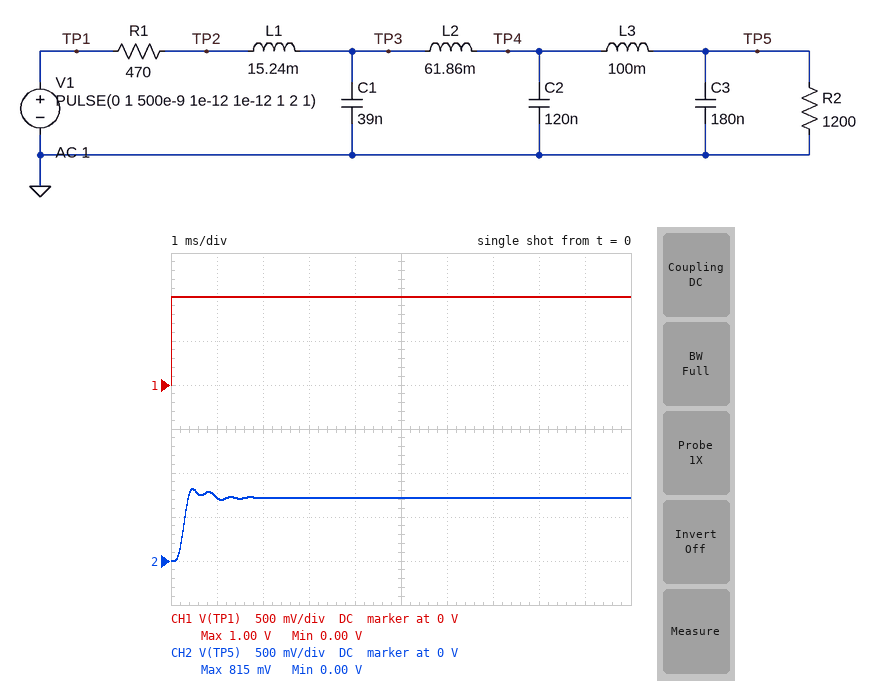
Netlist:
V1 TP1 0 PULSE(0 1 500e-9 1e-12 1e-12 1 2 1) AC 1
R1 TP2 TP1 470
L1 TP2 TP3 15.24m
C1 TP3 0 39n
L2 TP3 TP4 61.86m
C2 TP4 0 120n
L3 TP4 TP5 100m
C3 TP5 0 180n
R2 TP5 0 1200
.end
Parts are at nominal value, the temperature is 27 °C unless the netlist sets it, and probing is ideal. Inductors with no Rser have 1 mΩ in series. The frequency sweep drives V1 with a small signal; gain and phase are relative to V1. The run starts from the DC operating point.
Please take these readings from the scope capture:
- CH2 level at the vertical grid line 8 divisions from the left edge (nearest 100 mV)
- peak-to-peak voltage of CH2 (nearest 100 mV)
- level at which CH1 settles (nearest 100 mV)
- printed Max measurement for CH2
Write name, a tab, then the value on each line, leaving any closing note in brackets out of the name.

CH2 level at the vertical grid line 8 divisions from the left edge	700 mV
peak-to-peak voltage of CH2	800 mV
level at which CH1 settles	1.0 V
printed Max measurement for CH2	815 mV
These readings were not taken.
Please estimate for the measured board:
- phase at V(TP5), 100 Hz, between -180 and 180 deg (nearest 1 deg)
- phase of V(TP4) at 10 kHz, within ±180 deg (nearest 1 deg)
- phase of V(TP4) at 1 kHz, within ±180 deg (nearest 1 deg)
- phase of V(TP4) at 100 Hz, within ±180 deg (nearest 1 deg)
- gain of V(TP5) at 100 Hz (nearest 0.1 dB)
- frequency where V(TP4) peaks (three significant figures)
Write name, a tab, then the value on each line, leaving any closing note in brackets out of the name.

phase at V(TP5), 100 Hz, between -180 and 180 deg	-8 deg
phase of V(TP4) at 10 kHz, within ±180 deg	43 deg
phase of V(TP4) at 1 kHz, within ±180 deg	-39 deg
phase of V(TP4) at 100 Hz, within ±180 deg	-5 deg
gain of V(TP5) at 100 Hz	-2.8 dB
frequency where V(TP4) peaks	2.32 kHz
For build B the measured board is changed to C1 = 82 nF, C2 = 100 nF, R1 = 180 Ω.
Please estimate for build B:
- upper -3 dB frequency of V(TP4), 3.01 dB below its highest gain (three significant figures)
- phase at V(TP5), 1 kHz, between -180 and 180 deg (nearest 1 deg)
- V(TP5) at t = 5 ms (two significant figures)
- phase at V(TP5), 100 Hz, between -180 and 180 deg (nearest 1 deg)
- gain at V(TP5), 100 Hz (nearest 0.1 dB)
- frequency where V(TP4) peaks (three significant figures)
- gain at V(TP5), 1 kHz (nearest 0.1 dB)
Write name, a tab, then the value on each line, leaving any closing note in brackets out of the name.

upper -3 dB frequency of V(TP4), 3.01 dB below its highest gain	2.71 kHz
phase at V(TP5), 1 kHz, between -180 and 180 deg	-108 deg
V(TP5) at t = 5 ms	870 mV
phase at V(TP5), 100 Hz, between -180 and 180 deg	-7 deg
gain at V(TP5), 100 Hz	-1.1 dB
frequency where V(TP4) peaks	2.52 kHz
gain at V(TP5), 1 kHz	0 dB
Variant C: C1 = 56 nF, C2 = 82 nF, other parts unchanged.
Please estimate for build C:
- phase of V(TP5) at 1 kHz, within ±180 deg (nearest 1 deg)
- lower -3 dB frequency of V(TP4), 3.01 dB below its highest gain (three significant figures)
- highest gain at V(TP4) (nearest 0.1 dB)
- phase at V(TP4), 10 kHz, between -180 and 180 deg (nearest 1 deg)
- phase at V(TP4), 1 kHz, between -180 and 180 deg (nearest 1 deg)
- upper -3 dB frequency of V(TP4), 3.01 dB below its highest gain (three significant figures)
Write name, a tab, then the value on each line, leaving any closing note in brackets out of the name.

phase of V(TP5) at 1 kHz, within ±180 deg	-98 deg
lower -3 dB frequency of V(TP4), 3.01 dB below its highest gain	2.38 kHz
highest gain at V(TP4)	6.3 dB
phase at V(TP4), 10 kHz, between -180 and 180 deg	36 deg
phase at V(TP4), 1 kHz, between -180 and 180 deg	-37 deg
upper -3 dB frequency of V(TP4), 3.01 dB below its highest gain	3.23 kHz
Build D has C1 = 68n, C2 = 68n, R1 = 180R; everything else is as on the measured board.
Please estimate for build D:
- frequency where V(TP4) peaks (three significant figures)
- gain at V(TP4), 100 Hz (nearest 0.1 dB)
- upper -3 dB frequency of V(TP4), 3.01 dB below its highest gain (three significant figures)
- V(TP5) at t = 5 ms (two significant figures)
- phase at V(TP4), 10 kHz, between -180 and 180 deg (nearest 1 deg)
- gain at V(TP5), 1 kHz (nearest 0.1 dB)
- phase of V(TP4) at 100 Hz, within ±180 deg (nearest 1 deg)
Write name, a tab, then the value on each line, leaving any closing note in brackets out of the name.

frequency where V(TP4) peaks	2.98 kHz
gain at V(TP4), 100 Hz	-1.2 dB
upper -3 dB frequency of V(TP4), 3.01 dB below its highest gain	3.19 kHz
V(TP5) at t = 5 ms	870 mV
phase at V(TP4), 10 kHz, between -180 and 180 deg	14 deg
gain at V(TP5), 1 kHz	-0.3 dB
phase of V(TP4) at 100 Hz, within ±180 deg	-3 deg
